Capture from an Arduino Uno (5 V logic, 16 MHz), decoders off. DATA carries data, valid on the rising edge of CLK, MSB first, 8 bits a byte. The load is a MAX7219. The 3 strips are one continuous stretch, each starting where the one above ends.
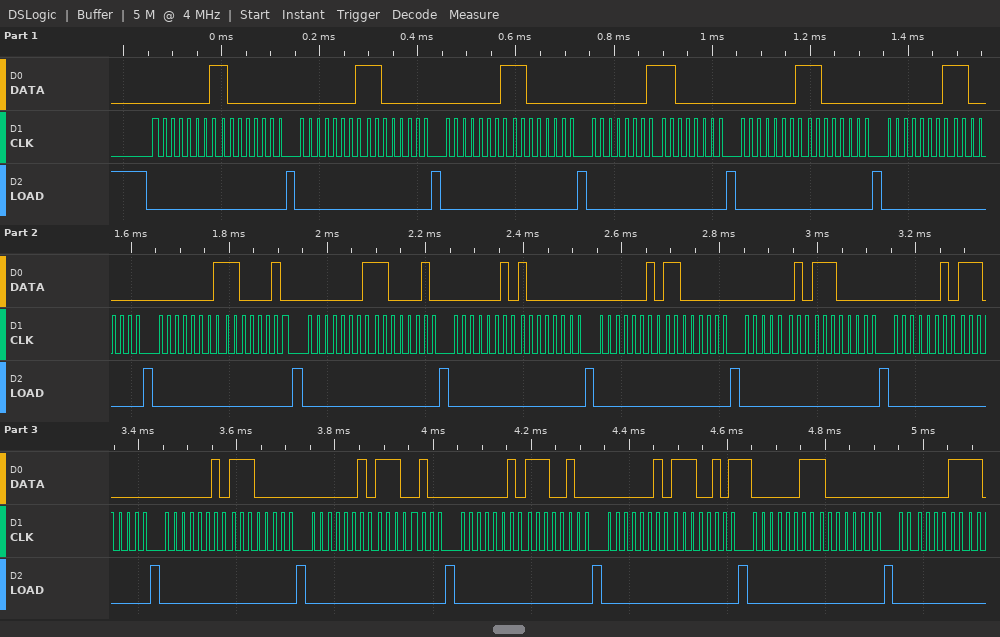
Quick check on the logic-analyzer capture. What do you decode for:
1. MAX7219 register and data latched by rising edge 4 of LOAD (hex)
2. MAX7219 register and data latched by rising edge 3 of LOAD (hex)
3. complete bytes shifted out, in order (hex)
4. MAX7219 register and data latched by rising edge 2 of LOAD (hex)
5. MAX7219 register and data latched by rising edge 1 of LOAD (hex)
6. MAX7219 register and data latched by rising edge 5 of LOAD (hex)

register 0x1, data 0xC0
register 0x1, data 0xC0
0x01 0x80 0x01 0xC0 0x01 0xC0 0x01 0xC0 0x01 0xC0 0x01 0xC0 0x01 0xC2 0x01 0xC2 0x02 0x80 0x02 0xC0 0x02 0xE0 0x02 0xE0 0x02 0xE0 0x02 0xE4 0x02 0xE4 0x02 0xE5 0x03 0x80 0x03
register 0x1, data 0xC0
register 0x1, data 0x80
register 0x1, data 0xC0
